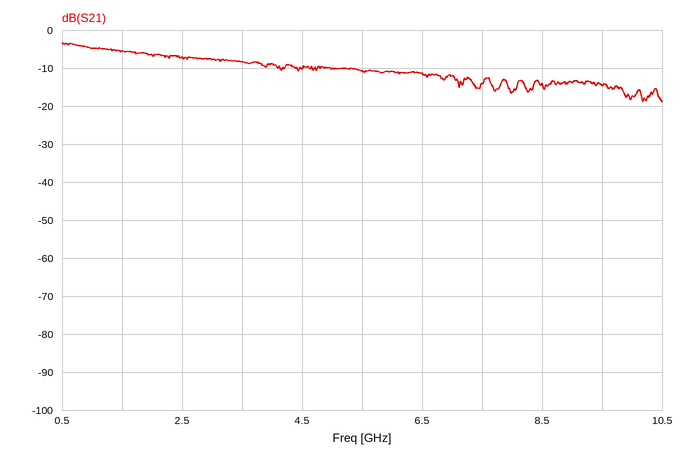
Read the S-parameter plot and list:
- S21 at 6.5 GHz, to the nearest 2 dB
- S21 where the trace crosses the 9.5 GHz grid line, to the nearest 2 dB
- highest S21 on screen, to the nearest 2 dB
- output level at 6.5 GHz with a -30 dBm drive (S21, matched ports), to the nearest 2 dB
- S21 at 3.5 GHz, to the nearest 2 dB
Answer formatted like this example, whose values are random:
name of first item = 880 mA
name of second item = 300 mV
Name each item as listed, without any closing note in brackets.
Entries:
S21 at 6.5 GHz, to the nearest 2 dB = -12 dB
S21 where the trace crosses the 9.5 GHz grid line, to the nearest 2 dB = -14 dB
highest S21 on screen, to the nearest 2 dB = -4 dB
output level at 6.5 GHz with a -30 dBm drive (S21, matched ports), to the nearest 2 dB = -42 dBm
S21 at 3.5 GHz, to the nearest 2 dB = -8 dB
